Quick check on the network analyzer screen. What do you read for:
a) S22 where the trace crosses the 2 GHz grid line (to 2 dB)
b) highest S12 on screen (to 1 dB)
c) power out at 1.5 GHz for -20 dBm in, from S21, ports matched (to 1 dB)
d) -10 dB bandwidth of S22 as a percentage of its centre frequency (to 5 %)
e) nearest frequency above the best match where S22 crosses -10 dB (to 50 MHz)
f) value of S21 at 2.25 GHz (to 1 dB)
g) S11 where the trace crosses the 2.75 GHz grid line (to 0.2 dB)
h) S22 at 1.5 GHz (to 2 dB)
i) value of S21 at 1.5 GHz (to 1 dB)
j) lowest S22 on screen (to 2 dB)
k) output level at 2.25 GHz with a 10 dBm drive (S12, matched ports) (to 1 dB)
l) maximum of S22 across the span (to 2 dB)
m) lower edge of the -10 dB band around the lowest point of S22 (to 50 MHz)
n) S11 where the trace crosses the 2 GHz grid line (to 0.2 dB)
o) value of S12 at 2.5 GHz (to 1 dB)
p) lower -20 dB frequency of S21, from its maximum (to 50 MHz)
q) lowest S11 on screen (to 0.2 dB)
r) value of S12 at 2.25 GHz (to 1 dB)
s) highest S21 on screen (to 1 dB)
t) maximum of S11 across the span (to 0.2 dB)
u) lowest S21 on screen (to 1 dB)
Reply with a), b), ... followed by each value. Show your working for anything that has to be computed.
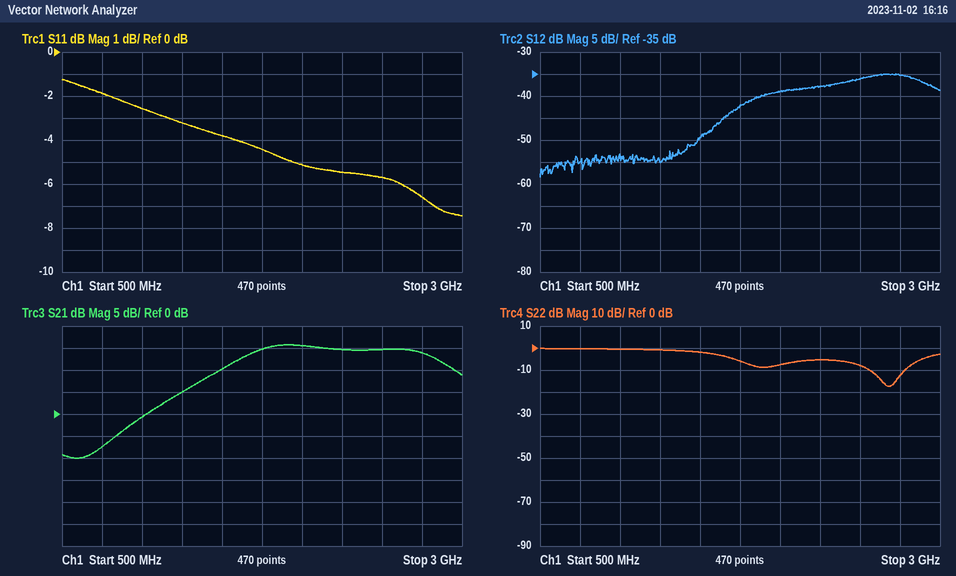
a) -8 dB
b) -35 dB
c) -20 dBm + (10 dB) = -10 dBm
d) 250 MHz / 2.675 GHz ≈ 9.35 %, so 10 % to the nearest 5 %
e) 2.80 GHz
f) 15 dB
g) -6.6 dB
h) -2 dB
i) 10 dB
j) -18 dB
k) 10 dBm + (-38 dB) = -28 dBm
l) 0 dB
m) 2.55 GHz
n) -5.2 dB
o) -36 dB
p) 850 MHz
q) -7.4 dB
r) -38 dB
s) 16 dB
t) -1.2 dB
u) -10 dB
